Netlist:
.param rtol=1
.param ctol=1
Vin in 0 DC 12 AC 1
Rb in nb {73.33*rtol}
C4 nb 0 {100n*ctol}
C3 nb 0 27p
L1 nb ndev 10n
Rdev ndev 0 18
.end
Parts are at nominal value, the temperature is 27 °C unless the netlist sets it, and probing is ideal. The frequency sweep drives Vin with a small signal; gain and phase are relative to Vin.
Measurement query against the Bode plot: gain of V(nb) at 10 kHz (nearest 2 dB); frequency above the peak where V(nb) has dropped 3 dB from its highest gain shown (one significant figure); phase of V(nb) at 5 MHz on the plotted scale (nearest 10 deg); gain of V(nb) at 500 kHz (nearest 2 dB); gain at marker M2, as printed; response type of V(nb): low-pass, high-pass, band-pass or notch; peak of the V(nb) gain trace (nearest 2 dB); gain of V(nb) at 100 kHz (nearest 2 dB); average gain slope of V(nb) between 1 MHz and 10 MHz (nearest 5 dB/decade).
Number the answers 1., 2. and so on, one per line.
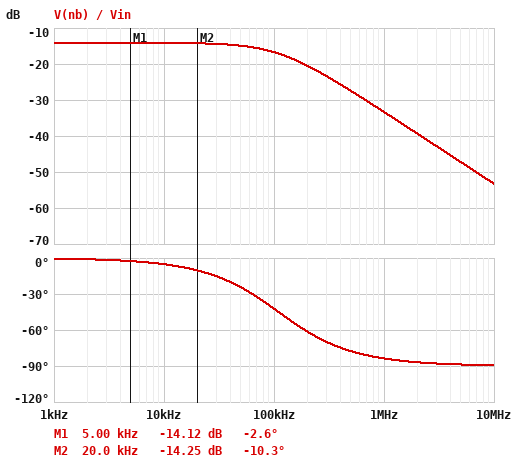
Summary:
1. -14 dB
2. 100 kHz
3. -90 deg
4. -28 dB
5. -14.25 dB
6. low-pass
7. -14 dB
8. -16 dB
9. -20 dB/decade
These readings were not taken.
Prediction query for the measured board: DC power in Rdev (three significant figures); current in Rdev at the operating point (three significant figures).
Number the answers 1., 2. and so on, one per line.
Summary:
1. 311 mW
2. 131 mA
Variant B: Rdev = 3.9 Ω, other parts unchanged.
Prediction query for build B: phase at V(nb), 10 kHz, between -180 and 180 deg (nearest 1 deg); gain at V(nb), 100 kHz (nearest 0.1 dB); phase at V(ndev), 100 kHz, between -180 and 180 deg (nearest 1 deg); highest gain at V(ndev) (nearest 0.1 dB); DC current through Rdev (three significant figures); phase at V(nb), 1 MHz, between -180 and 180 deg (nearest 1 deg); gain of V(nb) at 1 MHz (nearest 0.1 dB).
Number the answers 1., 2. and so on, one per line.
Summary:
1. -1 deg
2. -26.2 dB
3. -13 deg
4. -25.9 dB
5. 155 mA
6. -67 deg
7. -34.0 dB
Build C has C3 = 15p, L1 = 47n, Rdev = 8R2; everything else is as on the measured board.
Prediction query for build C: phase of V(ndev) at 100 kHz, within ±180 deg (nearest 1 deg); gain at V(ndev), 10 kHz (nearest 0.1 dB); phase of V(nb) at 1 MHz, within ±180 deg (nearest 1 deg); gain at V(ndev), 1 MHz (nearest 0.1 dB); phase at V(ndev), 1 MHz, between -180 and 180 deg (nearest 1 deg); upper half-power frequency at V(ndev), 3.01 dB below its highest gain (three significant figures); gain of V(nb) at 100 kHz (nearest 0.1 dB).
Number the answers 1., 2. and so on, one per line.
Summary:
1. -25 deg
2. -20.0 dB
3. -78 deg
4. -33.4 dB
5. -80 deg
6. 217 kHz
7. -20.8 dB
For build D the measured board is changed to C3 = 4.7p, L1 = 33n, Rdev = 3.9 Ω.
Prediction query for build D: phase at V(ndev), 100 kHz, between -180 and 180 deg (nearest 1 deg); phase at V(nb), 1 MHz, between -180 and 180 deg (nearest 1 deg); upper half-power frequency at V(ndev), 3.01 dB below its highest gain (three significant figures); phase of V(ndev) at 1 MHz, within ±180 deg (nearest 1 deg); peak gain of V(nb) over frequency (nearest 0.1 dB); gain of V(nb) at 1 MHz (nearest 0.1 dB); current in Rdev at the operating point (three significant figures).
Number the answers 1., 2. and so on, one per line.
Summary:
1. -13 deg
2. -66 deg
3. 439 kHz
4. -69 deg
5. -25.9 dB
6. -33.8 dB
7. 155 mA
